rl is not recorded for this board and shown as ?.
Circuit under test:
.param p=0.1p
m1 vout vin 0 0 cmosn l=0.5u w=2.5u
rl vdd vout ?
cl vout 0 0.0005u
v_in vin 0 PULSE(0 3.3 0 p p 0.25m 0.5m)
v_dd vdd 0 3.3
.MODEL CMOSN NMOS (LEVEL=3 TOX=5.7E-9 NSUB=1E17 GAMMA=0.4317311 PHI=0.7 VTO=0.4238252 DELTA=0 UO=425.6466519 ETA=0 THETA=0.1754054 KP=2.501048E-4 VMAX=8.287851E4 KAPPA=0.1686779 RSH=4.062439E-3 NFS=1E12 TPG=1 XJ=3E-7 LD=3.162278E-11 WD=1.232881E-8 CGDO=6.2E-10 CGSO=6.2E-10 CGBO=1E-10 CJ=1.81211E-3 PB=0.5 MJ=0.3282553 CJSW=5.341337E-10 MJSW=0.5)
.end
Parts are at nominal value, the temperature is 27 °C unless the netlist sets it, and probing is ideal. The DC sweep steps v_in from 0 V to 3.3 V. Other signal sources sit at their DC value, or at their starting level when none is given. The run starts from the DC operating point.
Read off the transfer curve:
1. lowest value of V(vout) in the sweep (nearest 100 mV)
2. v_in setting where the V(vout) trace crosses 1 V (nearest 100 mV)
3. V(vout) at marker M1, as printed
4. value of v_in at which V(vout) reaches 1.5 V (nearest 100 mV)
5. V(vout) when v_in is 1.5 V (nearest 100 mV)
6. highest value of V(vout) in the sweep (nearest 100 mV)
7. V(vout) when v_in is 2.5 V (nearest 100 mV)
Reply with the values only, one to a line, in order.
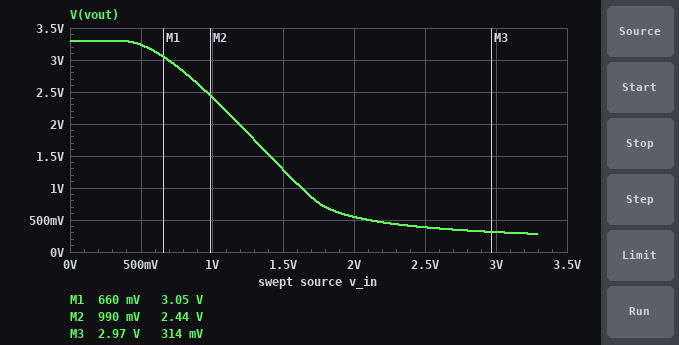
300 mV
1.6 V
3.05 V
1.4 V
1.3 V
3.3 V
400 mV
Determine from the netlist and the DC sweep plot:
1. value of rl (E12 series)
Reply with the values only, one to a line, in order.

5.6 kΩ
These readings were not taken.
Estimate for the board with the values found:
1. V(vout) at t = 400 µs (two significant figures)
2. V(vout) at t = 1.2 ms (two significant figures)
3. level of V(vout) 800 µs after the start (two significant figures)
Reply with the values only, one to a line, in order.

3.3 V
280 mV
3.3 V
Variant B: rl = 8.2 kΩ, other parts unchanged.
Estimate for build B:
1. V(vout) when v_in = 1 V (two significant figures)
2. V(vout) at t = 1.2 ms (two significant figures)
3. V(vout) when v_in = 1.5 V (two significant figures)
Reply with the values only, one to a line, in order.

2.0 V
180 mV
590 mV
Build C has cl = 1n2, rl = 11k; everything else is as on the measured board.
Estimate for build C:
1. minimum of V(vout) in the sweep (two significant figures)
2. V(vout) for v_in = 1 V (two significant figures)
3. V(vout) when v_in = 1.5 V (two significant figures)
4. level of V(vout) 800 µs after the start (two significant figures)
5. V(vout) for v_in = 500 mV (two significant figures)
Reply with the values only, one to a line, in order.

130 mV
1.6 V
360 mV
3.2 V
3.2 V
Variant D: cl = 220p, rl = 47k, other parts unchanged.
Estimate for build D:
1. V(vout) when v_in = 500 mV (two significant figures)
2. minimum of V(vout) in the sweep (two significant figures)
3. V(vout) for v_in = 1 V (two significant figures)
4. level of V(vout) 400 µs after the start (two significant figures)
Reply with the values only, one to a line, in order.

2.8 V
30 mV
120 mV
3.3 V
